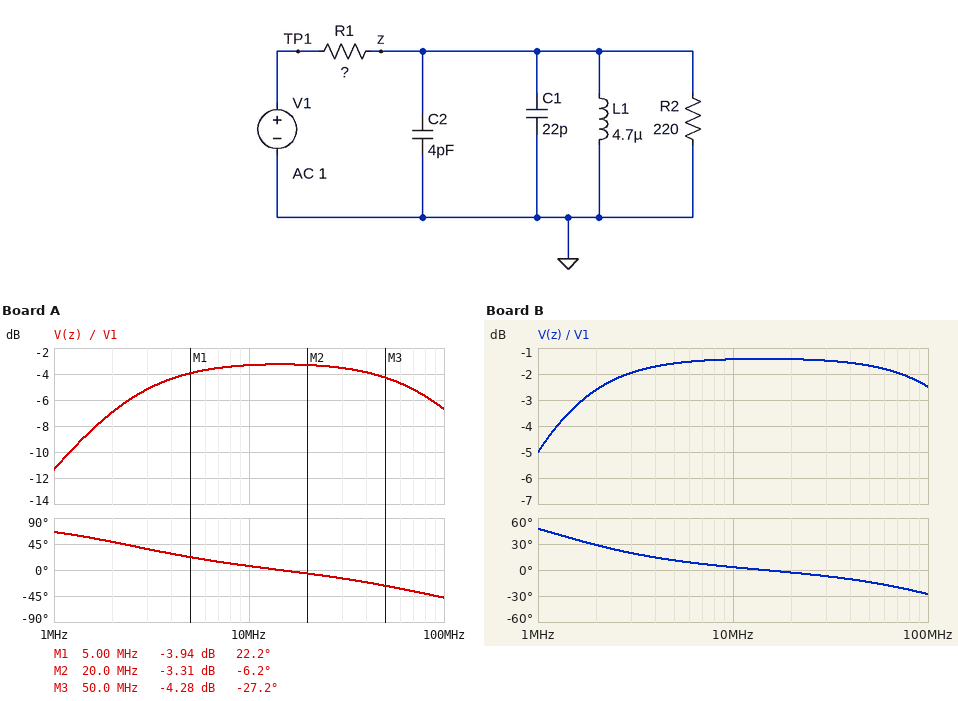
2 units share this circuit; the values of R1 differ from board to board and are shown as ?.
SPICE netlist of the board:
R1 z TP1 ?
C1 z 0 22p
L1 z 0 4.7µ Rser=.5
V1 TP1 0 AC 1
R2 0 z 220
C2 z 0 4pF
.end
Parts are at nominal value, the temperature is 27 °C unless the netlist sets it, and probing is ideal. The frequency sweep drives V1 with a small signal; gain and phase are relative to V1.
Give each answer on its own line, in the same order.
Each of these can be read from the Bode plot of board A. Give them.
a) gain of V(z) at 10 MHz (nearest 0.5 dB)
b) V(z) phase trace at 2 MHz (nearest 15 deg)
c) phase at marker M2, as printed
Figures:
-3.5 dB
45 deg
-6.2 deg
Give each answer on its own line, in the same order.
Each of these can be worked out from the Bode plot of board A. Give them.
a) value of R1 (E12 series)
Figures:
100 Ω
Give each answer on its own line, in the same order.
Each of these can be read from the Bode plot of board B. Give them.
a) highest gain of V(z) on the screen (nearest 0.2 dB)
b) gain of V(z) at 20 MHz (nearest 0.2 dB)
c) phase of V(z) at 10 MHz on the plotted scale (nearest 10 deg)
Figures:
-1.4 dB
-1.4 dB
0 deg
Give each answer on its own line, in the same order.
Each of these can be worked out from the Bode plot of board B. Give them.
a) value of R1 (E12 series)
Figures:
39 Ω
